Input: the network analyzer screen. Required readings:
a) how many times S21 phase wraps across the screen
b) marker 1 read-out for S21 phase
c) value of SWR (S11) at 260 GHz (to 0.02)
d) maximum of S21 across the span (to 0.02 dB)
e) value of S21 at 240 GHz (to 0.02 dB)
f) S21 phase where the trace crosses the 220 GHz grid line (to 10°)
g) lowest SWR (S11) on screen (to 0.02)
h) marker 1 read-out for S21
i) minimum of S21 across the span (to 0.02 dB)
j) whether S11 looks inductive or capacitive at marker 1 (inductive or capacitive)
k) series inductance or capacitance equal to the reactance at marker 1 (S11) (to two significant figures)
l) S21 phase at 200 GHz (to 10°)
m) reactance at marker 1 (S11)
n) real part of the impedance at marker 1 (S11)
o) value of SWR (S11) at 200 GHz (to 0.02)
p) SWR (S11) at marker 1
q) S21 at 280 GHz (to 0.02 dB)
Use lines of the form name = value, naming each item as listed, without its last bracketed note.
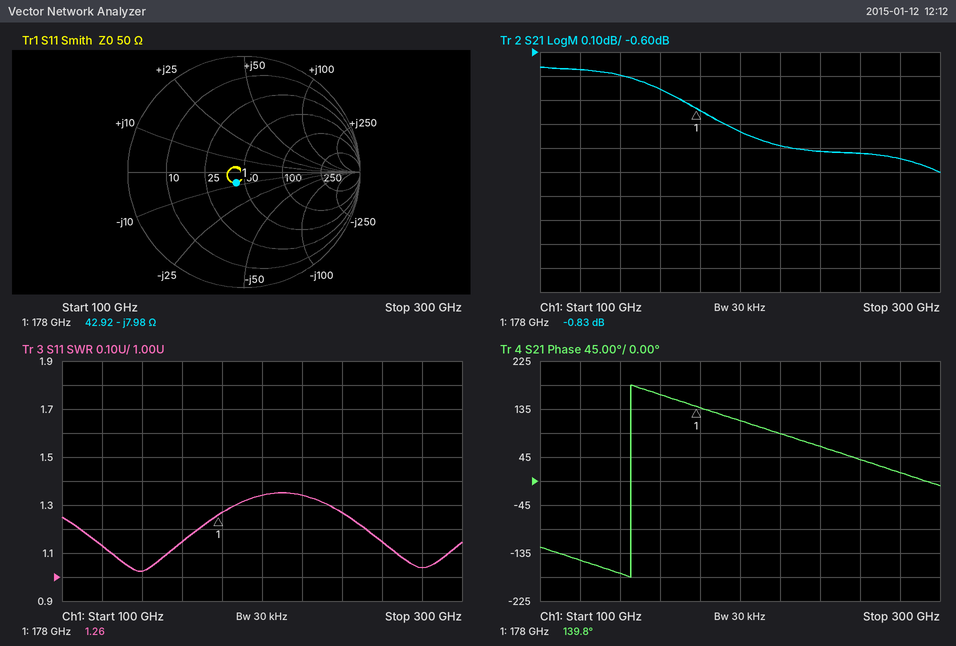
how many times S21 phase wraps across the screen = 1
marker 1 read-out for S21 phase = 139.8°
value of SWR (S11) at 260 GHz = 1.14
maximum of S21 across the span = -0.66 dB
value of S21 at 240 GHz = -1.02 dB
S21 phase where the trace crosses the 220 GHz grid line = 90°
lowest SWR (S11) on screen = 1.02
marker 1 read-out for S21 = -0.83 dB
minimum of S21 across the span = -1.10 dB
whether S11 looks inductive or capacitive at marker 1 = capacitive
series inductance or capacitance equal to the reactance at marker 1 (S11) = 110 fF
S21 phase at 200 GHz = 110°
reactance at marker 1 = -7.98 Ω
real part of the impedance at marker 1 = 42.92 Ω
value of SWR (S11) at 200 GHz = 1.34
SWR (S11) at marker 1 = 1.26
S21 at 280 GHz = -1.04 dB
